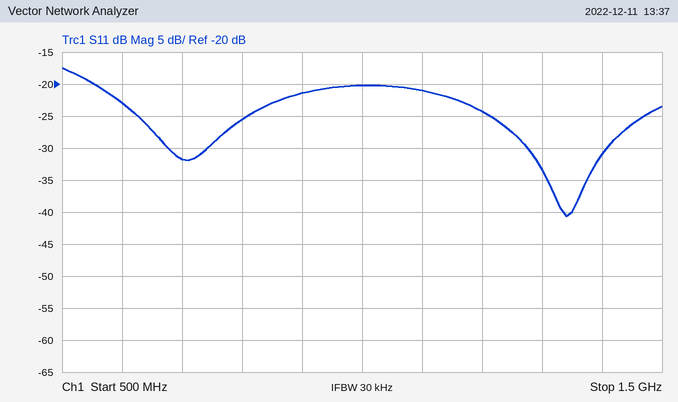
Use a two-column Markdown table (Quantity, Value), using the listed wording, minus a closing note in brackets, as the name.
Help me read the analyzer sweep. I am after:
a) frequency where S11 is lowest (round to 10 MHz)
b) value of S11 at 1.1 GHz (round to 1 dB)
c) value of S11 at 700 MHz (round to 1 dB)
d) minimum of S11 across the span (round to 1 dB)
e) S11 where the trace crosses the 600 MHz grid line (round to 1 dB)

| Quantity | Value |
|---|---|
| frequency where S11 is lowest | 1.34 GHz |
| value of S11 at 1.1 GHz | -21 dB |
| value of S11 at 700 MHz | -32 dB |
| minimum of S11 across the span | -41 dB |
| S11 where the trace crosses the 600 MHz grid line | -23 dB |
